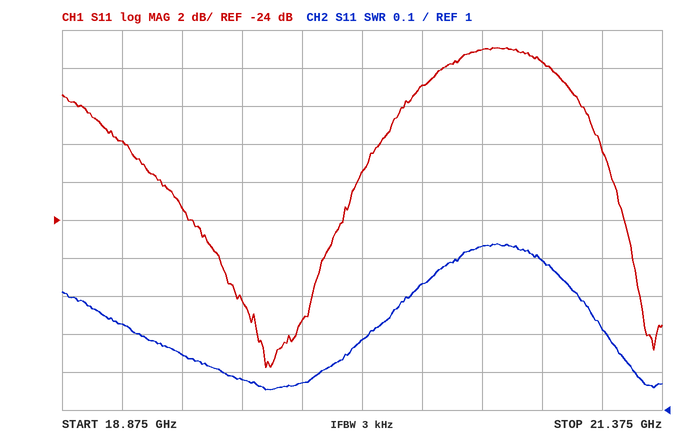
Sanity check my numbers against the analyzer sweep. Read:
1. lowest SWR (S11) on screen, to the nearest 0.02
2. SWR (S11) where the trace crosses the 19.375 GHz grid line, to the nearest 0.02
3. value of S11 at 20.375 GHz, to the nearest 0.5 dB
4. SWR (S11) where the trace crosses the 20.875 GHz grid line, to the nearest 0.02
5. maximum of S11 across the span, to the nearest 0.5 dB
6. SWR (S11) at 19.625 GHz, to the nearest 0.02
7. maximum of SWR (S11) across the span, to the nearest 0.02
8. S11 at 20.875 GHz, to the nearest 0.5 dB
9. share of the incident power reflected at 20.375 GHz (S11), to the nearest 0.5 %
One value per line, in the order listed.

1.06
1.14
-17.0 dB
1.40
-15.0 dB
1.08
1.44
-15.5 dB
2.0 %
